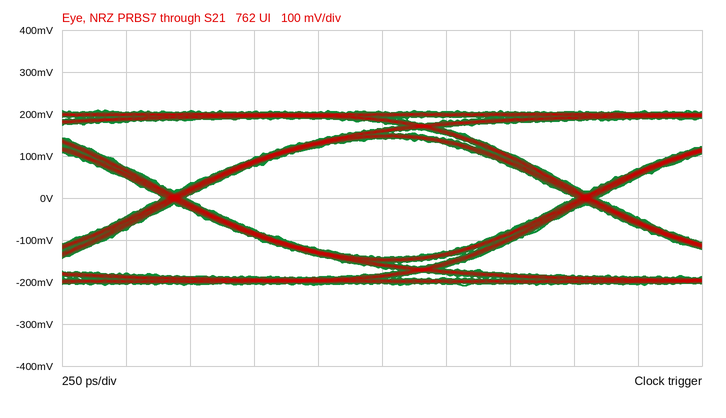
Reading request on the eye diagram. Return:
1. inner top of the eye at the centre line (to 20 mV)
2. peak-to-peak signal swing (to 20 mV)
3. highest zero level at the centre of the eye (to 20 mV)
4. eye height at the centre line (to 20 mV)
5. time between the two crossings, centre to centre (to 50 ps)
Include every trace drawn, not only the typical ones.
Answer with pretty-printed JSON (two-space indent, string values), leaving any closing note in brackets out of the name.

{
  "inner top of the eye at the centre line": "140 mV",
  "peak-to-peak signal swing": "420 mV",
  "highest zero level at the centre of the eye": "-140 mV",
  "eye height at the centre line": "280 mV",
  "time between the two crossings, centre to centre": "1.60 ns"
}
